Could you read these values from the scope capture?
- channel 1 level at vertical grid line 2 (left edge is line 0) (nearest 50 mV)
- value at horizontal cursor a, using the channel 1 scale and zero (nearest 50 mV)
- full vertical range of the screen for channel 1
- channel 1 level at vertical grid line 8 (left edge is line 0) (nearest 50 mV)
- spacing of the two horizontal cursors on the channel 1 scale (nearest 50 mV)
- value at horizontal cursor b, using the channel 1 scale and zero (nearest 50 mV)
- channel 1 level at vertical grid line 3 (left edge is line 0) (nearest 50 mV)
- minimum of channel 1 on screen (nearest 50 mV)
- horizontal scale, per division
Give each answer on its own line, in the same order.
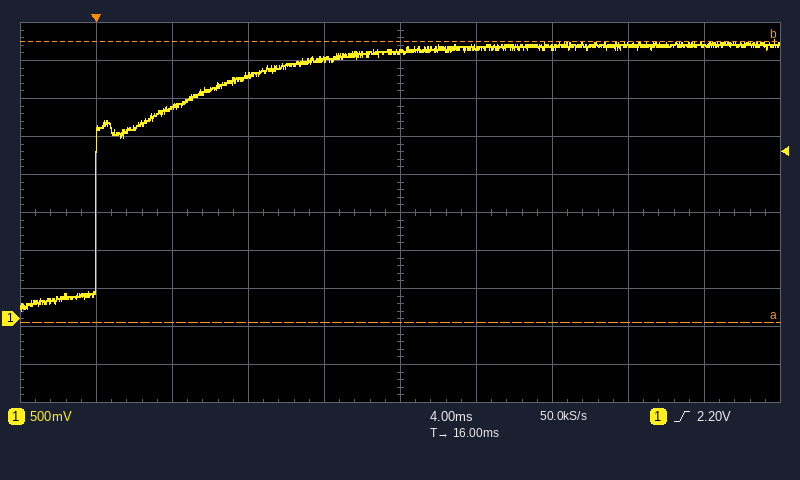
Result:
2.80 V
-50 mV
5 V
3.60 V
3.70 V
3.65 V
3.20 V
100 mV
4 ms
